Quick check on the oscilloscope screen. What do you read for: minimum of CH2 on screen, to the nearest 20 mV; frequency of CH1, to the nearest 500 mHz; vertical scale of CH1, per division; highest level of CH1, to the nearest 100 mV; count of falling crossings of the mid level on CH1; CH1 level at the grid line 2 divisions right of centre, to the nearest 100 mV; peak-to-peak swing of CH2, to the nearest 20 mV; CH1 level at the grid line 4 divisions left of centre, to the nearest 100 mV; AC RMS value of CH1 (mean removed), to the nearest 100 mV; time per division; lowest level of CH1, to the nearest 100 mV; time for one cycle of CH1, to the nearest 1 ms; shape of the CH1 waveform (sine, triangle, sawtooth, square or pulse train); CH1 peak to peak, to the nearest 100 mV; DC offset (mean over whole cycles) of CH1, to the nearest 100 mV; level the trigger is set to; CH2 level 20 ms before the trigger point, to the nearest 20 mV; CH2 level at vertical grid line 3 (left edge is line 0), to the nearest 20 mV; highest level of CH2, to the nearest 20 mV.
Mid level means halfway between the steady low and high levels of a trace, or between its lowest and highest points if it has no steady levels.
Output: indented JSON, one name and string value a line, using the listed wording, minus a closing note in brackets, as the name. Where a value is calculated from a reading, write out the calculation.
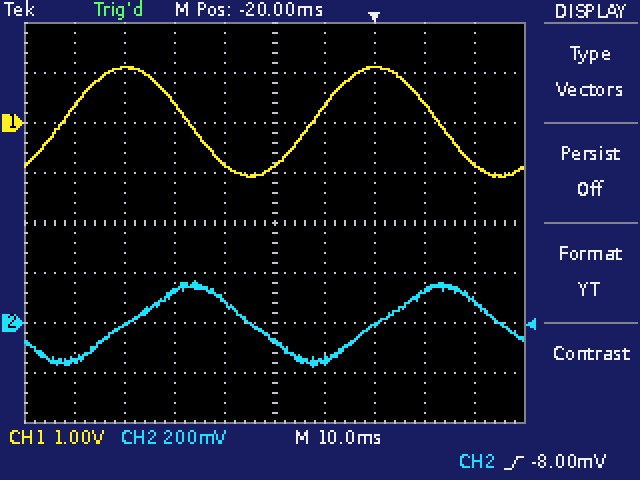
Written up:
{
  "minimum of CH2 on screen, to the nearest 20 mV": "-180 mV",
  "frequency of CH1, to the nearest 500 mHz": "1 / 50 ms ≈ 20.0 Hz",
  "vertical scale of CH1, per division": "1 V",
  "highest level of CH1, to the nearest 100 mV": "1.1 V",
  "count of falling crossings of the mid level on CH1": "2",
  "CH1 level at the grid line 2 divisions right of centre, to the nearest 100 mV": "1.1 V",
  "peak-to-peak swing of CH2, to the nearest 20 mV": "160 mV − (-180 mV) = 340 mV",
  "CH1 level at the grid line 4 divisions left of centre, to the nearest 100 mV": "300 mV",
  "AC RMS value of CH1 (mean removed), to the nearest 100 mV": "2.2 V / (2√2) ≈ 778 mV, so 800 mV to the nearest 100 mV",
  "time per division": "10 ms",
  "lowest level of CH1, to the nearest 100 mV": "-1.1 V",
  "time for one cycle of CH1, to the nearest 1 ms": "50 ms",
  "shape of the CH1 waveform": "sine",
  "CH1 peak to peak, to the nearest 100 mV": "1.1 V − (-1.1 V) = 2.2 V",
  "DC offset (mean over whole cycles) of CH1, to the nearest 100 mV": "(1.1 V + (-1.1 V)) / 2 ≈ 0.0 V",
  "level the trigger is set to": "-8.00 mV",
  "CH2 level 20 ms before the trigger point, to the nearest 20 mV": "-80 mV",
  "CH2 level at vertical grid line 3 (left edge is line 0), to the nearest 20 mV": "120 mV",
  "highest level of CH2, to the nearest 20 mV": "160 mV"
}
